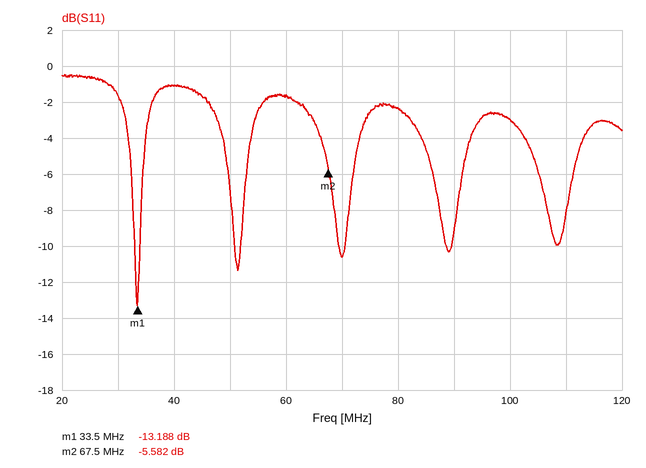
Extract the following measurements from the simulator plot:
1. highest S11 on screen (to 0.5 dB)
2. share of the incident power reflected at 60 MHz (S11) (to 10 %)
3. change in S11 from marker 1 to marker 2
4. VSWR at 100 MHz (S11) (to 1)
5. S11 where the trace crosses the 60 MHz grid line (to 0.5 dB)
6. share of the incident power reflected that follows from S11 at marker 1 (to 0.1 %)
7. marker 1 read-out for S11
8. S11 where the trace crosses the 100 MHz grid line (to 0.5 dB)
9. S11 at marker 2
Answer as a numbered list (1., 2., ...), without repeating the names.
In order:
1. -0.5 dB
2. 70 %
3. 7.606 dB
4. 6
5. -1.5 dB
6. 4.8 %
7. -13.188 dB
8. -3.0 dB
9. -5.582 dB
